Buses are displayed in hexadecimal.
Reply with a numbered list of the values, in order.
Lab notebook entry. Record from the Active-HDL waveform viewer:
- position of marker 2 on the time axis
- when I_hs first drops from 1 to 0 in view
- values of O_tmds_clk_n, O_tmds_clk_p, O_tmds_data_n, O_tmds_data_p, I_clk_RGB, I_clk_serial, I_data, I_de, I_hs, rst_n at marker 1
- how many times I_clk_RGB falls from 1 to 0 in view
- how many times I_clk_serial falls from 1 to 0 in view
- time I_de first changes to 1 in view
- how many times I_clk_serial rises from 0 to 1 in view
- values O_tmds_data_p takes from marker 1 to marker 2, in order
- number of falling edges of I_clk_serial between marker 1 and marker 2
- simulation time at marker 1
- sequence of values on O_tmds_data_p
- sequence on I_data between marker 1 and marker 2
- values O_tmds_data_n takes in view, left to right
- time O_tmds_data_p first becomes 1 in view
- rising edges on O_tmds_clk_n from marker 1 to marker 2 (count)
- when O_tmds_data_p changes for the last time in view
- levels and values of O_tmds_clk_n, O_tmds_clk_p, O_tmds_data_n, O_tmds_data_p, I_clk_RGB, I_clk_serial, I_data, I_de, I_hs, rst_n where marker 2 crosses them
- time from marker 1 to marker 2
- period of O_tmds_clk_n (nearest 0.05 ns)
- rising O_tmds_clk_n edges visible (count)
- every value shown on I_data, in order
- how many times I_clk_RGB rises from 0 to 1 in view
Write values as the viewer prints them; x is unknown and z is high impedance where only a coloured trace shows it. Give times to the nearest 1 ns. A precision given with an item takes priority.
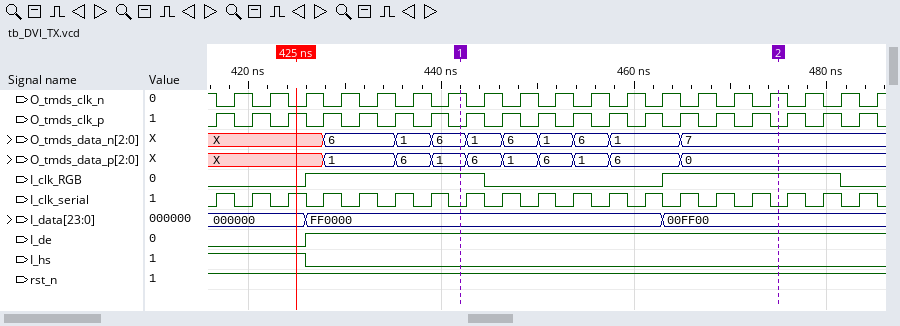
1. 475 ns
2. 426 ns
3. O_tmds_clk_n=1, O_tmds_clk_p=0, O_tmds_data_n=6, O_tmds_data_p=1, I_clk_RGB=1, I_clk_serial=0, I_data=FF0000, I_de=1, I_hs=0, rst_n=1
4. 2
5. 19
6. 426 ns
7. 19
8. 1, 6, 1, 6, 1, 6, 0
9. 9
10. 442 ns
11. X, 1, 6, 1, 6, 1, 6, 1, 6, 0
12. FF0000, 00FF00
13. X, 6, 1, 6, 1, 6, 1, 6, 1, 7
14. 428 ns
15. 9
16. 465 ns
17. O_tmds_clk_n=1, O_tmds_clk_p=0, O_tmds_data_n=7, O_tmds_data_p=0, I_clk_RGB=1, I_clk_serial=0, I_data=00FF00, I_de=1, I_hs=0, rst_n=1
18. 33 ns
19. 3.7 ns
20. 19
21. 000000, FF0000, 00FF00
22. 2
